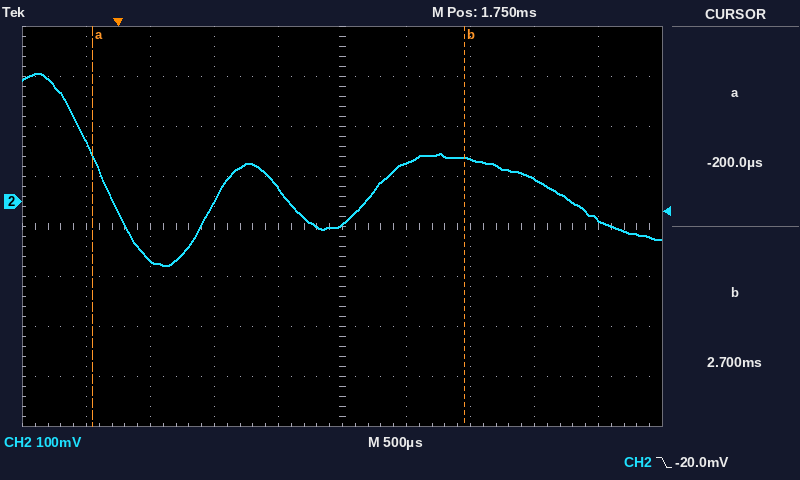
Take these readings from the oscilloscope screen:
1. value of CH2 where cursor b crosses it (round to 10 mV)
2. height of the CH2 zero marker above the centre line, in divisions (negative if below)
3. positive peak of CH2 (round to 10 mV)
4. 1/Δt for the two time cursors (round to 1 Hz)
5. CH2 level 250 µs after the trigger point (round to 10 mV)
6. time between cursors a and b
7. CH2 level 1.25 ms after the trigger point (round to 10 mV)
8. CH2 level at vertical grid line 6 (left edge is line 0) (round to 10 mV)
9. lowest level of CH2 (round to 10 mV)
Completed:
90 mV
+0.5 div
260 mV
345 Hz
-120 mV
2.90 ms
30 mV
80 mV
-130 mV
